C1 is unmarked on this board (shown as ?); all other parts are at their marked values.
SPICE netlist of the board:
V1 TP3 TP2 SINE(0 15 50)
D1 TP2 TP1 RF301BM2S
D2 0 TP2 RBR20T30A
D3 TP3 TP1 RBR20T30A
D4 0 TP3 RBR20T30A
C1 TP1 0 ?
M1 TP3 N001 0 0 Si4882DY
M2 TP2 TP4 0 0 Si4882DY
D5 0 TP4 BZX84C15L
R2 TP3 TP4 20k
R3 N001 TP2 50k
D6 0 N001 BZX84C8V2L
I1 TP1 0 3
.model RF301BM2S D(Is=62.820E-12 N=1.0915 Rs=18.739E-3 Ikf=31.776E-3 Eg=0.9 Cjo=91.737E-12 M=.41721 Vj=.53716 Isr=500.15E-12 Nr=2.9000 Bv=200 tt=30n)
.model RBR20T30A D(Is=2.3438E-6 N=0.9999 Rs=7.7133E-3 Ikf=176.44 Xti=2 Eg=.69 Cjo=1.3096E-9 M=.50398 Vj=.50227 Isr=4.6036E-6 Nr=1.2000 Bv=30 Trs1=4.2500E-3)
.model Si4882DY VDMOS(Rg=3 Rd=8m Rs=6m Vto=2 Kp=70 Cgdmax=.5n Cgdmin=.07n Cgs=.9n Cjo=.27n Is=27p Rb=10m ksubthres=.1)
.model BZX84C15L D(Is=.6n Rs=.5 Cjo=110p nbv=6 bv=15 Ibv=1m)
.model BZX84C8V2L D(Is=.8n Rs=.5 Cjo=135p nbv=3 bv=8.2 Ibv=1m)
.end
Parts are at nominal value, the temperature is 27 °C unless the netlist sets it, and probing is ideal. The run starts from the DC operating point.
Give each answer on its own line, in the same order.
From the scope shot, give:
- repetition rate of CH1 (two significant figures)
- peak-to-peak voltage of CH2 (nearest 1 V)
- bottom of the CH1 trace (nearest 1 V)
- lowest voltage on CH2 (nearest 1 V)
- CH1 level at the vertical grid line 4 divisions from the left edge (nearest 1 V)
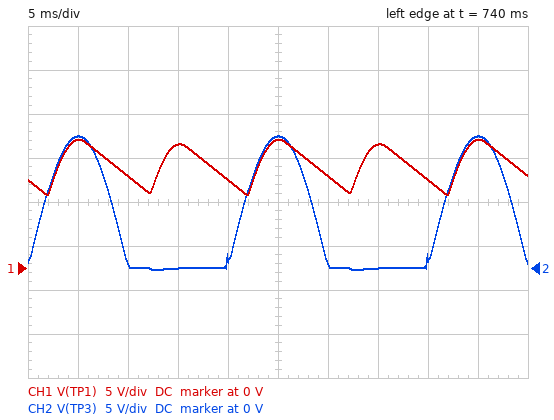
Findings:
100 Hz
15 V
8 V
0 V
10 V
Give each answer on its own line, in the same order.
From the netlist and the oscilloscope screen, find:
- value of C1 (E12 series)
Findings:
3.3 mF
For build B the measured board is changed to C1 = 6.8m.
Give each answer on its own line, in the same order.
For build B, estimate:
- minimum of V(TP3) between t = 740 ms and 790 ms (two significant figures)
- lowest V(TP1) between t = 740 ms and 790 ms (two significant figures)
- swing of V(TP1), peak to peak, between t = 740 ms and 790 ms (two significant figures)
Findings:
-270 mV
11 V
3.7 V
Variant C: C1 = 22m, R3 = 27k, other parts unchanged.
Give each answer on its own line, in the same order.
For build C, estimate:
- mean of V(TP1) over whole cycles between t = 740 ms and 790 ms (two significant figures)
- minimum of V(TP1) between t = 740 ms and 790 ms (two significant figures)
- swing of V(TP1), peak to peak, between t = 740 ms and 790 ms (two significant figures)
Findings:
14 V
13 V
1.6 V
